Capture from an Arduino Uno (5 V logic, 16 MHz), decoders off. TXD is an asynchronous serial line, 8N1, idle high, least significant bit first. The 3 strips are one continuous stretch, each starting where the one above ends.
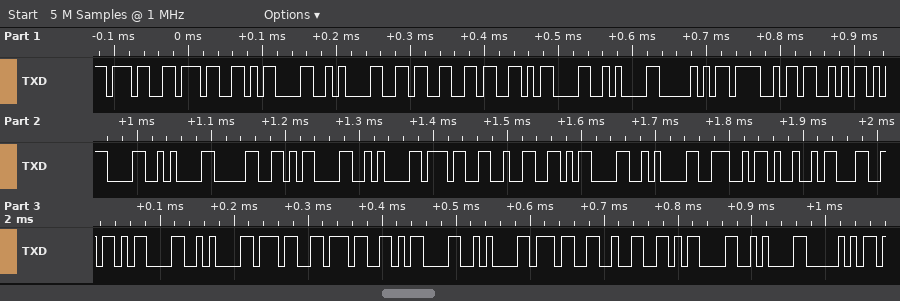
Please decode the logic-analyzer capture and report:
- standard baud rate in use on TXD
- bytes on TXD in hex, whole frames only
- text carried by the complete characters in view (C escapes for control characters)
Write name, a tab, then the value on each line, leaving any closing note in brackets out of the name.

standard baud rate in use on TXD	115200 baud
bytes on TXD in hex, whole frames only	37 37 0D 0A 36 36 0D 0A 50 4F 53 0D 0A 30 0D 0A 37 32 0D 0A 4E 49 4C 0D 0A 37 37 0D 0A 37 32 0D 0A 50
text carried by the complete characters in view	"77\r\n66\r\nPOS\r\n0\r\n72\r\nNIL\r\n77\r\n72\r\nP"
